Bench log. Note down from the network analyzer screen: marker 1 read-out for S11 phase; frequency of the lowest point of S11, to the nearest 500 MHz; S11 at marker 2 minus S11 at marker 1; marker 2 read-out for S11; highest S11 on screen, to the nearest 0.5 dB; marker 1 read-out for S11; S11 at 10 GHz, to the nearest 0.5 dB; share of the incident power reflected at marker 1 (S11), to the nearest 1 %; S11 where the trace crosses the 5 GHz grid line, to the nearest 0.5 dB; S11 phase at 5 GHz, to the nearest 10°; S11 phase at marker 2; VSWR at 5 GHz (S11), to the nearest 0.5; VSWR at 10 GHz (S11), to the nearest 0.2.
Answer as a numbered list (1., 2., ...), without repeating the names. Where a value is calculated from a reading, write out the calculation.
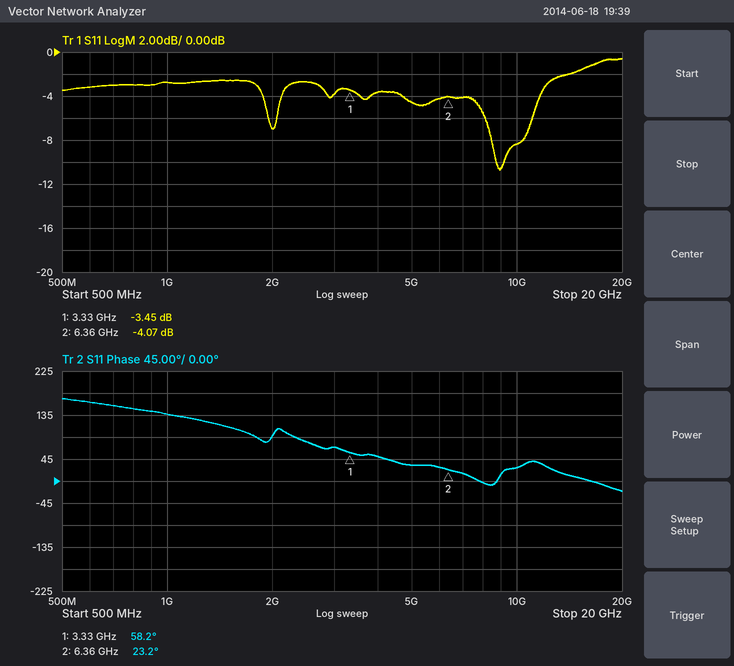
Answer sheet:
1. 58.2°
2. 9.0 GHz
3. -4.07 − (-3.45) = -0.62 dB
4. -4.07 dB
5. -0.5 dB
6. -3.45 dB
7. -8.5 dB
8. 10^(-3.45/10) ≈ 45 %
9. -4.5 dB
10. 30°
11. 23.2°
12. |Γ| = 10^(-4.5/20) = 0.5957; VSWR = (1 + 0.5957)/(1 − 0.5957) ≈ 4.0
13. |Γ| = 10^(-8.5/20) = 0.3758; VSWR = (1 + 0.3758)/(1 − 0.3758) ≈ 2.2
